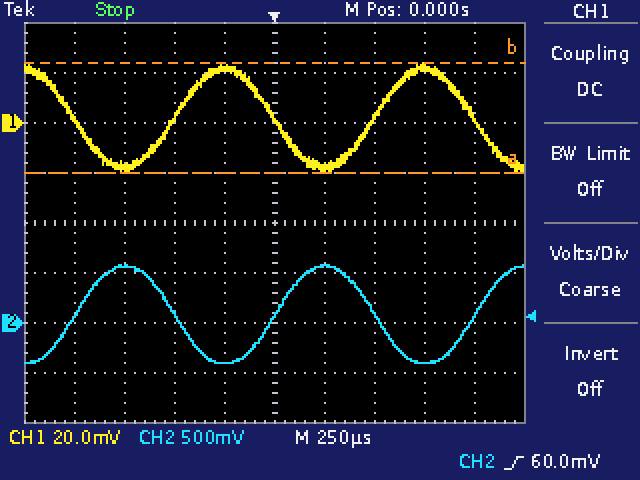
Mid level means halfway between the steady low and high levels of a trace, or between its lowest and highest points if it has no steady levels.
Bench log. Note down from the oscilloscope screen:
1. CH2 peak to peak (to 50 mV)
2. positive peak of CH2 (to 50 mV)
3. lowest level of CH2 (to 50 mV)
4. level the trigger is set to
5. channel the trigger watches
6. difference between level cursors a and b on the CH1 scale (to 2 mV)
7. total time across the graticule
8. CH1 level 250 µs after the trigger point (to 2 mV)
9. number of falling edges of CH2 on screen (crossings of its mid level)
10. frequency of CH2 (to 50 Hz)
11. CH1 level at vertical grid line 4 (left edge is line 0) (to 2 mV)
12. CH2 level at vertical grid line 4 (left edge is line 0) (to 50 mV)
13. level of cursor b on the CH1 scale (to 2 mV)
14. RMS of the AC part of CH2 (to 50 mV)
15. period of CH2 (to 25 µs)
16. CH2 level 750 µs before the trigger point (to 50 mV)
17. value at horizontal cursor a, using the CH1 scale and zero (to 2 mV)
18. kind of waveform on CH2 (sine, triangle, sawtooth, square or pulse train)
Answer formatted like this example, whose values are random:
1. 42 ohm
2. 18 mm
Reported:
1. 1.00 V
2. 600 mV
3. -400 mV
4. 60.0 mV
5. CH2
6. 44 mV
7. 2.5 ms
8. -18 mV
9. 2
10. 1.00 kHz
11. 22 mV
12. -400 mV
13. 24 mV
14. 350 mV
15. 1.000 ms
16. 550 mV
17. -20 mV
18. sine
